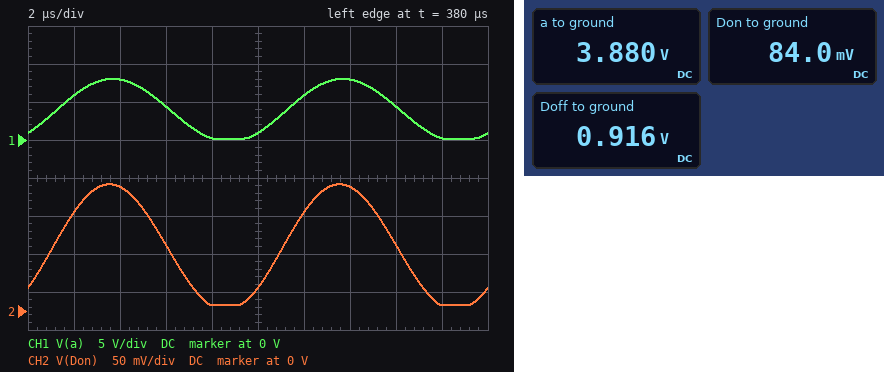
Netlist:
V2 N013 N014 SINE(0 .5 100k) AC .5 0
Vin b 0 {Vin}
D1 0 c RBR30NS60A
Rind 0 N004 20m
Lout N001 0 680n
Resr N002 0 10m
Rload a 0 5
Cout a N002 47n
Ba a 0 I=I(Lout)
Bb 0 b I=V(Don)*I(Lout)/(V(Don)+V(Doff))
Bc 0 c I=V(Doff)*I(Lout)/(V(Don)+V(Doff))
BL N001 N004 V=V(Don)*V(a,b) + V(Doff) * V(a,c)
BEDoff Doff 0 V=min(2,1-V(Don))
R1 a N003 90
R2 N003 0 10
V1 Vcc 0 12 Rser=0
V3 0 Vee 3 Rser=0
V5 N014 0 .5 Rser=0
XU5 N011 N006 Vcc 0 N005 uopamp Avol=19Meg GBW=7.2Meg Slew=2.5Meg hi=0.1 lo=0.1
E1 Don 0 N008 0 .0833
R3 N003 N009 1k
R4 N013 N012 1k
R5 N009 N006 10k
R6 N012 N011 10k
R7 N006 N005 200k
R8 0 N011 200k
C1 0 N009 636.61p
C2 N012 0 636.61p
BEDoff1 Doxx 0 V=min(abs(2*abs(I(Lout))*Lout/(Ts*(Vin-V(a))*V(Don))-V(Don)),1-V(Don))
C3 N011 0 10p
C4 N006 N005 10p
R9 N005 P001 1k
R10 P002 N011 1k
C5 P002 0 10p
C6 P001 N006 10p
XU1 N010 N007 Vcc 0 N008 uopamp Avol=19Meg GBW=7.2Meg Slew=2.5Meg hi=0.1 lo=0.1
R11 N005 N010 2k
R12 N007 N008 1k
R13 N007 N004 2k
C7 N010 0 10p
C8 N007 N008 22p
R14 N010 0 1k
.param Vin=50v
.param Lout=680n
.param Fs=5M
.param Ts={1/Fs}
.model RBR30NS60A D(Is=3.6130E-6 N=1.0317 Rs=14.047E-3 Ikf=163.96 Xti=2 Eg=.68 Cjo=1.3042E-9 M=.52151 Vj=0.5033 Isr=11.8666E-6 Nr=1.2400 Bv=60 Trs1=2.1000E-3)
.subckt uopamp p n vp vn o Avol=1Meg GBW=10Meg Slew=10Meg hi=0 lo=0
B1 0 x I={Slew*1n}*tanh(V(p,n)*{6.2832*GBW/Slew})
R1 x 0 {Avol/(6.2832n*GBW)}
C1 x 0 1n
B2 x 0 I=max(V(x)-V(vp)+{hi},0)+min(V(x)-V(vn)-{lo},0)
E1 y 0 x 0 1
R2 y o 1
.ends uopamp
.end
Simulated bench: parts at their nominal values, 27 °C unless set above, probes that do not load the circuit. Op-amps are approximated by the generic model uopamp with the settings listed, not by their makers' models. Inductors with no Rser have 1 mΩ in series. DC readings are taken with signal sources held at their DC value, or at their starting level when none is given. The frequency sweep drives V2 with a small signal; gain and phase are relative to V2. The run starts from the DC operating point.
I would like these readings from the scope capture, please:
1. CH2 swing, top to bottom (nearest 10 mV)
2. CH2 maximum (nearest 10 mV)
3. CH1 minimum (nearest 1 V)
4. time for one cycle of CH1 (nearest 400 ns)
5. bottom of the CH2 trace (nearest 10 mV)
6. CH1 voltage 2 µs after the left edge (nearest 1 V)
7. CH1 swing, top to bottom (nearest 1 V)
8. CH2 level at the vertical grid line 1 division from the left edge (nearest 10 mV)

160 mV
170 mV
0 V
10.0 µs
10 mV
6 V
8 V
130 mV
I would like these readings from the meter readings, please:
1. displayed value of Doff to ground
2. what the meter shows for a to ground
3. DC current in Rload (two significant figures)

0.916 V
3.880 V
780 mA
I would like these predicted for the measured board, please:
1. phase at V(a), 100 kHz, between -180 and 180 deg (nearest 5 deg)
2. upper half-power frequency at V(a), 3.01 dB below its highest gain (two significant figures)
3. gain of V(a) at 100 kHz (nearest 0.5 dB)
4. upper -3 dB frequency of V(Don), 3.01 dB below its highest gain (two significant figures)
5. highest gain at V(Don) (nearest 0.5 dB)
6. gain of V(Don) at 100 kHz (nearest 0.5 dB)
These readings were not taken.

-45 deg
250 kHz
18.5 dB
240 kHz
-15.5 dB
-15.5 dB
